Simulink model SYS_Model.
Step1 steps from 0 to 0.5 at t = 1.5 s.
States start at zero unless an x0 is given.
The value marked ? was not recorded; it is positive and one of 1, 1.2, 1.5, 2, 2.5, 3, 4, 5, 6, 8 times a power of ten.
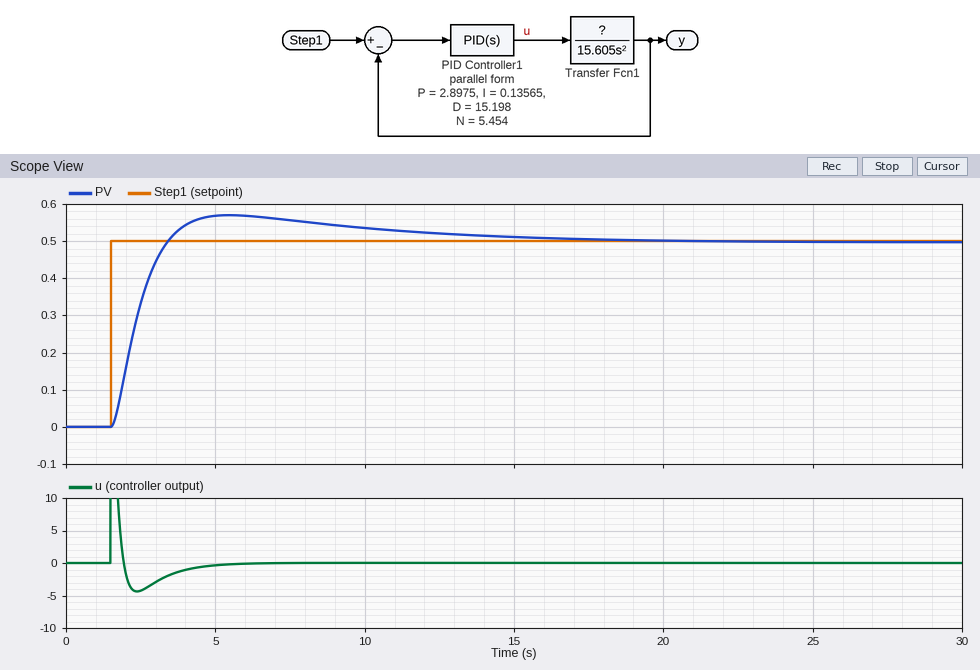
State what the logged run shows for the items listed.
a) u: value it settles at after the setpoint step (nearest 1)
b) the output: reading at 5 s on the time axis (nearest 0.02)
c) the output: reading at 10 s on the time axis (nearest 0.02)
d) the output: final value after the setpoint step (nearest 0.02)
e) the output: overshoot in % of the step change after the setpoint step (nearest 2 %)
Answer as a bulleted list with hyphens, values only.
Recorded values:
- 0
- 0.56
- 0.54
- 0.50
- 14 %
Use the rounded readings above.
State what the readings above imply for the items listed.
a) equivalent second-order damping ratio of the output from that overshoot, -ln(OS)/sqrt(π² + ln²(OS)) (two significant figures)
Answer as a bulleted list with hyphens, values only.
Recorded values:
- 0.53
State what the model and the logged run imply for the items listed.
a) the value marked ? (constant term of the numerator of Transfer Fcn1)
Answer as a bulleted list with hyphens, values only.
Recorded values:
- 1
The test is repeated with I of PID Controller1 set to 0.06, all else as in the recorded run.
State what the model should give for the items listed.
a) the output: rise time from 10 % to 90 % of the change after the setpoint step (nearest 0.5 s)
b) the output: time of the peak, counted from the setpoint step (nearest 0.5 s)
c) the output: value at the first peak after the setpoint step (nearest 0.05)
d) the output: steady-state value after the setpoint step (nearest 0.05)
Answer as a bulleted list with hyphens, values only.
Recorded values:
- 1.5 s
- 4.0 s
- 0.55
- 0.50
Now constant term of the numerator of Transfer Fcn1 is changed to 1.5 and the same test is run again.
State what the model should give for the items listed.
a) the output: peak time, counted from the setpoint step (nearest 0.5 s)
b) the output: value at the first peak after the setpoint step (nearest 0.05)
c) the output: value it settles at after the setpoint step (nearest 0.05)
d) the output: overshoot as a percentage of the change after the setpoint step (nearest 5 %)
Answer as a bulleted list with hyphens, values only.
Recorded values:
- 2.5 s
- 0.55
- 0.50
- 10 %
